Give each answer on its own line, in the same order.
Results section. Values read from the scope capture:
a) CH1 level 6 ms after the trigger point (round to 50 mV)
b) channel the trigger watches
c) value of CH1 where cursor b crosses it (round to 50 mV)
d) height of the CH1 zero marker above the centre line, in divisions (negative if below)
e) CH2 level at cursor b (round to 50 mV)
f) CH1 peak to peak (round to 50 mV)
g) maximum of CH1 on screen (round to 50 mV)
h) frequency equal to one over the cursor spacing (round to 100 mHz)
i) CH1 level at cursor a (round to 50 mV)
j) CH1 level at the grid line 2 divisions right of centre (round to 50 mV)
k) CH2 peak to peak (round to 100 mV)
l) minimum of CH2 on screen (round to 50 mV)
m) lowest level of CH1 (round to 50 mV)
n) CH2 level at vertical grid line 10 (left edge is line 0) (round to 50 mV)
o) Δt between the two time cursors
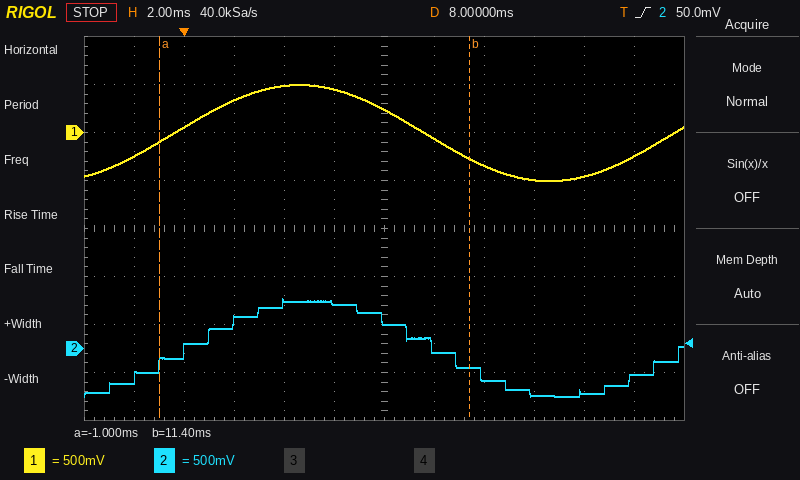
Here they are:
450 mV
CH2
-250 mV
+2.0 div
-200 mV
1.00 V
500 mV
80.6 Hz
-100 mV
-350 mV
1.00 V
-500 mV
-500 mV
-450 mV
12.4 ms
